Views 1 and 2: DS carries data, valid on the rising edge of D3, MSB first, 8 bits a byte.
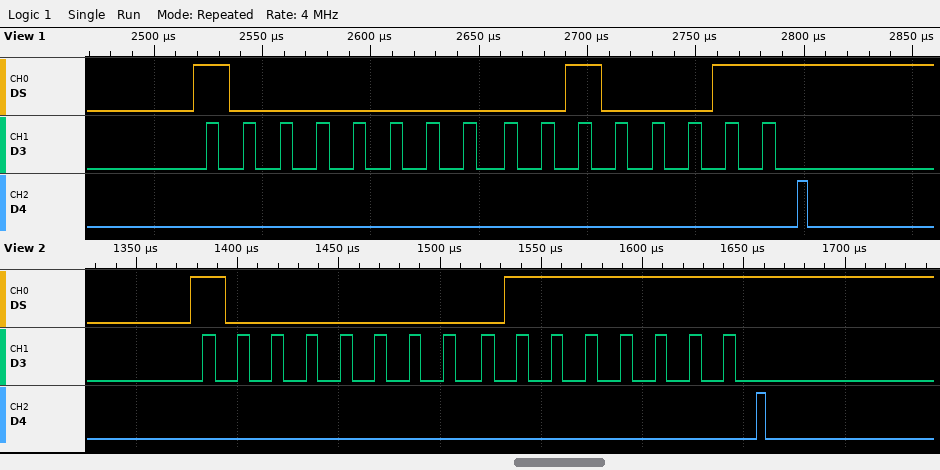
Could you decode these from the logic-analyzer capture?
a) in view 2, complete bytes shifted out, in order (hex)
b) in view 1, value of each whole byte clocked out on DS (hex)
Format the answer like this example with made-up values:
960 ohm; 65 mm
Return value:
80 7F; 80 23
